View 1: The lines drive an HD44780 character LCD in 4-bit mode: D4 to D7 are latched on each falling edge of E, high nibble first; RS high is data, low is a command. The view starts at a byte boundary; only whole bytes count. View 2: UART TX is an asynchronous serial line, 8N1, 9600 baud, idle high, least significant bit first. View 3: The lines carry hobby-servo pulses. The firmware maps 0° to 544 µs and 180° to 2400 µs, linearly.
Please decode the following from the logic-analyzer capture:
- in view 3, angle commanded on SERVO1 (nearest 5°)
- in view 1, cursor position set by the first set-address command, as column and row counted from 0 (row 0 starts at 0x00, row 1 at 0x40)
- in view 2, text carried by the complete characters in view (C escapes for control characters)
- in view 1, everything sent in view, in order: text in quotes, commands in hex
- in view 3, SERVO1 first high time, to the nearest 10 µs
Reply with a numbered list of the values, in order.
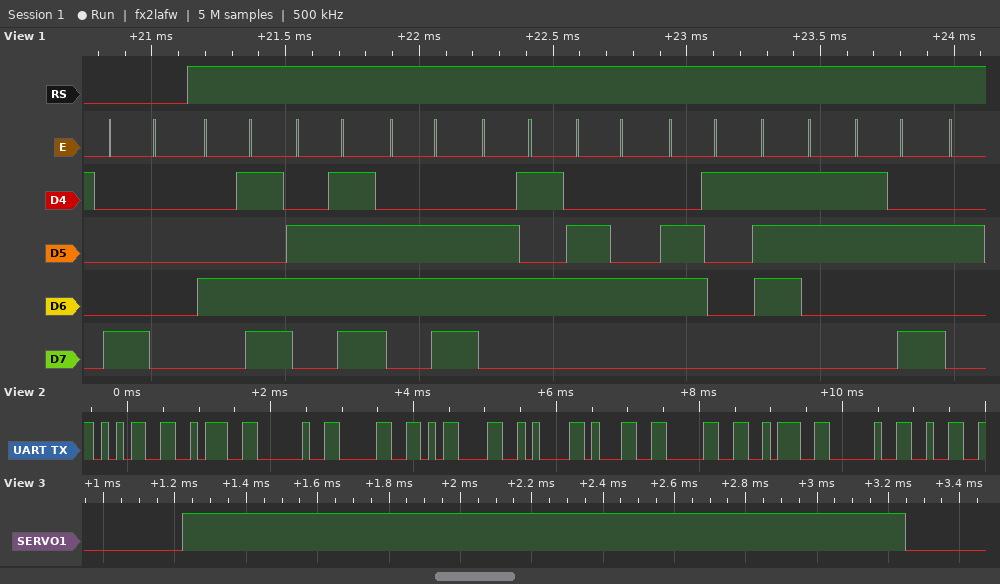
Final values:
1. 145°
2. column 0, row 0
3. "5: 0\r\n10: 2"
4. 0x80 "Monedas:"
5. 2030 µs
